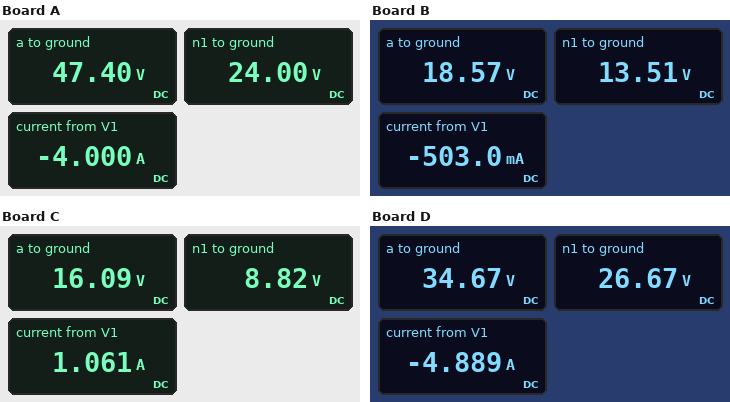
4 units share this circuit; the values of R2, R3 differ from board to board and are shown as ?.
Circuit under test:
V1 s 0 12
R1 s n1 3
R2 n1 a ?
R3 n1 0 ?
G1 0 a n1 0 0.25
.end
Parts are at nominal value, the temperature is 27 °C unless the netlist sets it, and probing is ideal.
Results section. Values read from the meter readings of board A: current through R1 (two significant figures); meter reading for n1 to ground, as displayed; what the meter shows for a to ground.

4.0 A
24.00 V
47.40 V
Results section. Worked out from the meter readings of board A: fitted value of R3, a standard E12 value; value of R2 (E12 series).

12 Ω
3.9 Ω
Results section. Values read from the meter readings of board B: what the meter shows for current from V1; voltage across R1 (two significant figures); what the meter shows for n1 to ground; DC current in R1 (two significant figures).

-503.0 mA
1.5 V
13.51 V
500 mA
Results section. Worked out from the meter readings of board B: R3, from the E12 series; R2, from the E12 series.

4.7 Ω
1.5 Ω
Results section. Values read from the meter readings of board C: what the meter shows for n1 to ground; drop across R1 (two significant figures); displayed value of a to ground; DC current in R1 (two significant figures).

8.82 V
3.2 V
16.09 V
1.1 A
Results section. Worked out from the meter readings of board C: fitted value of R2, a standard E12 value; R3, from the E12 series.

3.3 Ω
2.7 Ω
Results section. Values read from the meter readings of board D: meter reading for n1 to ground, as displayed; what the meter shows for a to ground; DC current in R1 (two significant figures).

26.67 V
34.67 V
4.9 A
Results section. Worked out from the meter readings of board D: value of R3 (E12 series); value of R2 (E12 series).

15 Ω
1.2 Ω
